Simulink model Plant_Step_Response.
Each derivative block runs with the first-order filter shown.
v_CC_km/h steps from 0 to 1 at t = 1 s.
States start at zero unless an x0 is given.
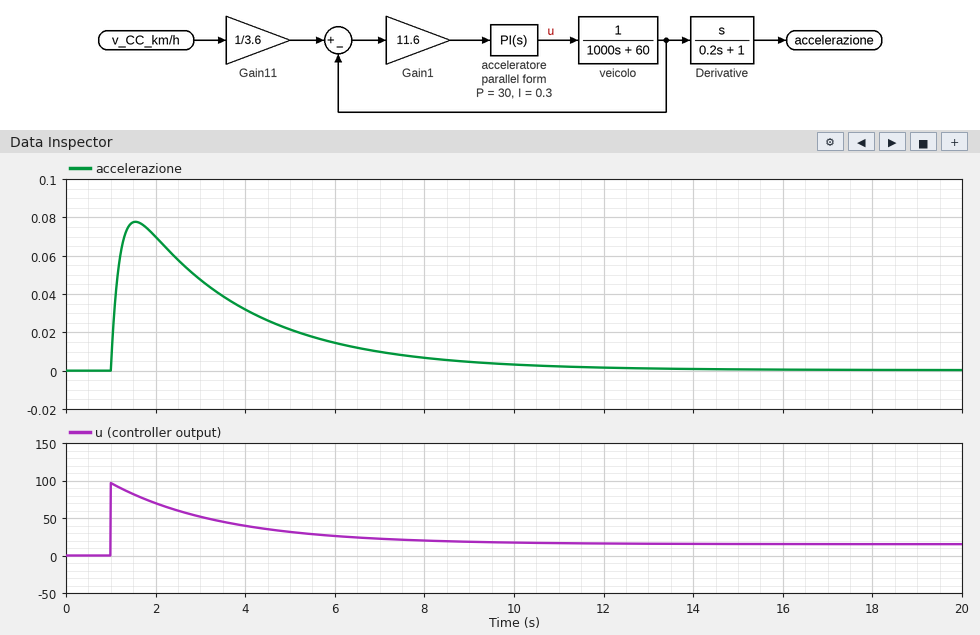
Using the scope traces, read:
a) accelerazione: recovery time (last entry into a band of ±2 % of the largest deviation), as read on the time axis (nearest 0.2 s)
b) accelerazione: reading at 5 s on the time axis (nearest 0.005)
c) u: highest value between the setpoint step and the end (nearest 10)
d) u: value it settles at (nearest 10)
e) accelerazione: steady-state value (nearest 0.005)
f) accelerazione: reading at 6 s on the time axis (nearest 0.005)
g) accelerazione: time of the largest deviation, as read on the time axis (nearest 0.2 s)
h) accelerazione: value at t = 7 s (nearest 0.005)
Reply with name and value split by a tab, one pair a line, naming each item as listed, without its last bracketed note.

accelerazione: recovery time (last entry into a band of ±2 % of the largest deviation), as read on the time axis	11.8 s
accelerazione: reading at 5 s on the time axis	0.020
u: highest value between the setpoint step and the end	100
u: value it settles at	20
accelerazione: steady-state value	0.000
accelerazione: reading at 6 s on the time axis	0.015
accelerazione: time of the largest deviation, as read on the time axis	1.6 s
accelerazione: value at t = 7 s	0.010
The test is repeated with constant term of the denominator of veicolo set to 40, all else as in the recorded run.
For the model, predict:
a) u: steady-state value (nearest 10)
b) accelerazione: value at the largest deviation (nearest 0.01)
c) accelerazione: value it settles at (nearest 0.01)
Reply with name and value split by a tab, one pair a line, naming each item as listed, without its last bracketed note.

u: steady-state value	10
accelerazione: value at the largest deviation	0.08
accelerazione: value it settles at	0.00
